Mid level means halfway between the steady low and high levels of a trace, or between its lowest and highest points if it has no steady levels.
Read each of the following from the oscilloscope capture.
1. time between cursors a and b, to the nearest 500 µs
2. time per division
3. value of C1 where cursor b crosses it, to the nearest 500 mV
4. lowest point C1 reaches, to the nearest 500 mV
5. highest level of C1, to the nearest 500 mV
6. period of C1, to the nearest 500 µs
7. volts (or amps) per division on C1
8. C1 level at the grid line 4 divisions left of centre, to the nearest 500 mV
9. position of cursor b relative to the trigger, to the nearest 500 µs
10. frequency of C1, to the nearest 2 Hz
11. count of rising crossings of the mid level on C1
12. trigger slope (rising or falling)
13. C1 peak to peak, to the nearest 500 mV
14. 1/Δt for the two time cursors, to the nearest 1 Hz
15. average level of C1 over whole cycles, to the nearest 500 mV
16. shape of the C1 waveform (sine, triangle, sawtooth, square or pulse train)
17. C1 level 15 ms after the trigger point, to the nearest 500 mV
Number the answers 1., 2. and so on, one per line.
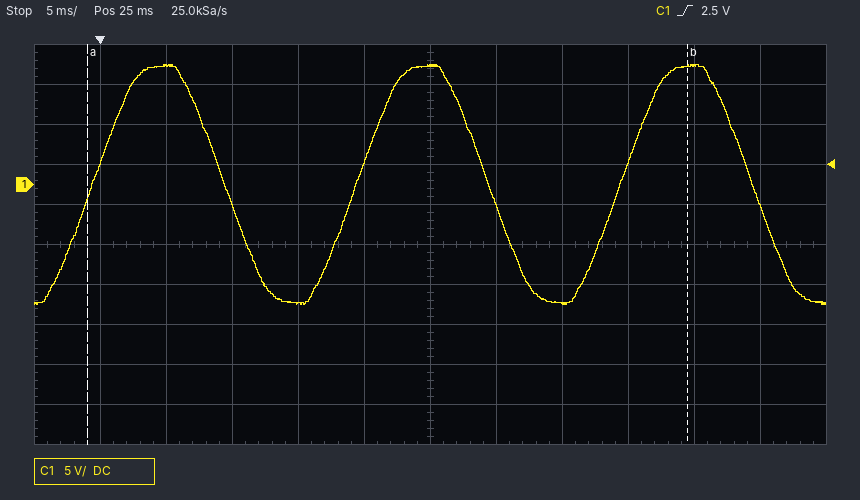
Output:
1. 45.5 ms
2. 5 ms
3. 15.0 V
4. -15.0 V
5. 15.0 V
6. 20.0 ms
7. 5 V
8. 15.0 V
9. +44.5 ms
10. 50 Hz
11. 3
12. rising
13. 30.0 V
14. 22 Hz
15. 0.0 V
16. sine
17. -15.0 V
